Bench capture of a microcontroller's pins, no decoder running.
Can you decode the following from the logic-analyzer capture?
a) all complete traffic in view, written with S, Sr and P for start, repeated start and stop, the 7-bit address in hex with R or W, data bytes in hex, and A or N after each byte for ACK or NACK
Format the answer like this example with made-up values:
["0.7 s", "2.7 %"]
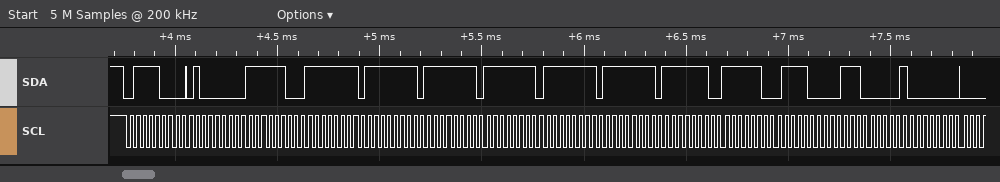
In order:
["S 3CW A 40 A FC A FF A FF A FF A FF A FF A FF A FE A FC A F0 A E0 A 80 A"]
